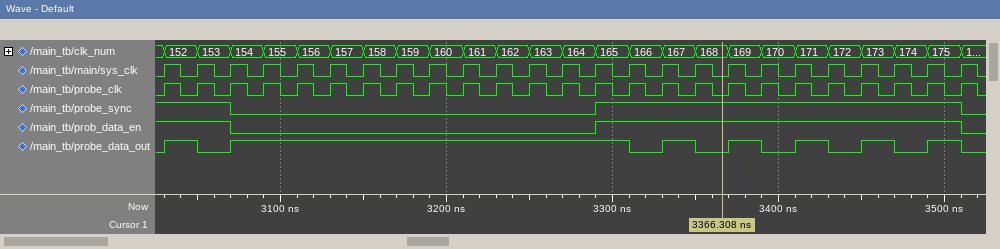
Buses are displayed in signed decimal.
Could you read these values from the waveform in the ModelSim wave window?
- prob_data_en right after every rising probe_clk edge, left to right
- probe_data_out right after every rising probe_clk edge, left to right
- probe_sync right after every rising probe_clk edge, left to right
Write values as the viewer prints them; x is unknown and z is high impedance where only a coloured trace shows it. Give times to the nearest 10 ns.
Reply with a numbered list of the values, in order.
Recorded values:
1. 1 1 0 0 0 0 0 0 0 0 0 0 0 1 1 1 1 1 1 1 1 1 1 1 0
2. 1 0 1 1 1 1 1 1 1 1 1 1 1 1 0 1 0 1 0 1 0 1 0 1 0
3. 1 1 0 0 0 0 0 0 0 0 0 0 0 1 1 1 1 1 1 1 1 1 1 1 0
